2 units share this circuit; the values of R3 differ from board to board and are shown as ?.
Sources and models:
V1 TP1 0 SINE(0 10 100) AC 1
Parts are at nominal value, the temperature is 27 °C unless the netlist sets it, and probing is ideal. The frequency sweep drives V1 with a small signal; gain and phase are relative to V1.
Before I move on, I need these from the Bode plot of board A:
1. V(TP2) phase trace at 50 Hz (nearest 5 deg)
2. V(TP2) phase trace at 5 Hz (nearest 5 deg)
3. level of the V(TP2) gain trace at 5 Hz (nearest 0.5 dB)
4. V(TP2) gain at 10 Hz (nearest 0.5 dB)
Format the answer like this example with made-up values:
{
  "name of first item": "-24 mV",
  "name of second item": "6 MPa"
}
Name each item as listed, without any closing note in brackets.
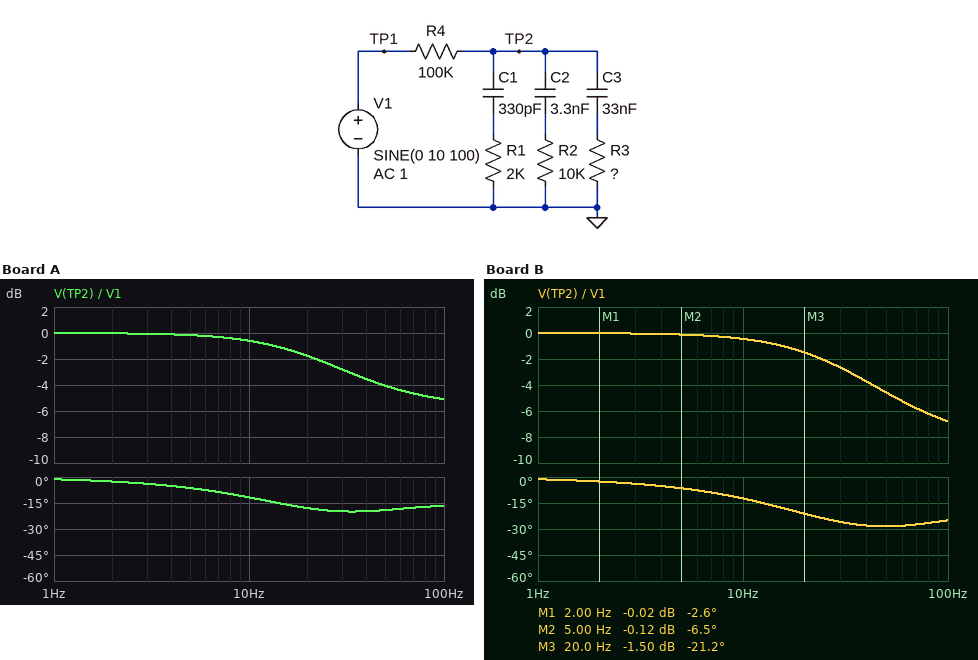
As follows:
{
  "V(TP2) phase trace at 50 Hz": "-20 deg",
  "V(TP2) phase trace at 5 Hz": "-5 deg",
  "level of the V(TP2) gain trace at 5 Hz": "0 dB",
  "V(TP2) gain at 10 Hz": "-0.5 dB"
}
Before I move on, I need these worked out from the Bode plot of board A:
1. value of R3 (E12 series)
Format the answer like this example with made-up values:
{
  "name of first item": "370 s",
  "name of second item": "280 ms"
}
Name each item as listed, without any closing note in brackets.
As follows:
{
  "value of R3": "120 kΩ"
}
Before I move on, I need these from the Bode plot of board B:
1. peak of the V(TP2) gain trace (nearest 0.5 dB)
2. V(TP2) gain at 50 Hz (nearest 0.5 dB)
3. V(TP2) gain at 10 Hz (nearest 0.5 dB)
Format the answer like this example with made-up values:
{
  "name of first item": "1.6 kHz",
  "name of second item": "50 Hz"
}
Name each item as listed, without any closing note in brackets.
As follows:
{
  "peak of the V(TP2) gain trace": "0 dB",
  "V(TP2) gain at 50 Hz": "-4.5 dB",
  "V(TP2) gain at 10 Hz": "-0.5 dB"
}
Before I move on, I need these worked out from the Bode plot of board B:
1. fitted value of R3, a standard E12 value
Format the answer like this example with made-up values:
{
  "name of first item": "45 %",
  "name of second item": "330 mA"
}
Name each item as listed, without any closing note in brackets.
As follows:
{
  "fitted value of R3, a standard E12 value": "68 kΩ"
}
